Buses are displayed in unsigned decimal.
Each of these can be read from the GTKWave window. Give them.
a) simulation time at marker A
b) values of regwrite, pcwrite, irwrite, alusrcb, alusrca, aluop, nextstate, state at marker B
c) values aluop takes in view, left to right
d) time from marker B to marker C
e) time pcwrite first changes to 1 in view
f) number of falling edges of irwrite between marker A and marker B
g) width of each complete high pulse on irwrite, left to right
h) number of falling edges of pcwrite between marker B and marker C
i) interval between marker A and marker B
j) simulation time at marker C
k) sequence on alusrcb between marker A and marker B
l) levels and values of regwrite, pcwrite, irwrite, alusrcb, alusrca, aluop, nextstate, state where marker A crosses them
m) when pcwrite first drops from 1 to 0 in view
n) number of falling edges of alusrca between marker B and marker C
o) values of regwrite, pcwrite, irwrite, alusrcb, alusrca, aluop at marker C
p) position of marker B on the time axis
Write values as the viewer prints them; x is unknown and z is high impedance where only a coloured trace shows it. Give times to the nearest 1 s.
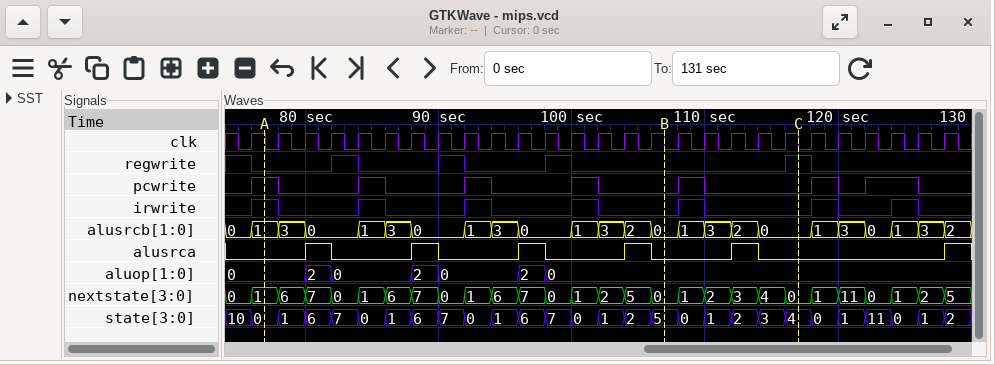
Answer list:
77 s
regwrite=0, pcwrite=0, irwrite=0, alusrcb=0, alusrca=0, aluop=0, nextstate=0, state=5
0, 2, 0, 2, 0, 2, 0
10 s
76 s
4
2 s, 2 s, 2 s, 2 s, 2 s, 2 s, 2 s
1
30 s
117 s
1, 3, 0, 1, 3, 0, 1, 3, 0, 1, 3, 2, 0
regwrite=0, pcwrite=1, irwrite=1, alusrcb=1, alusrca=0, aluop=0, nextstate=1, state=0
78 s
1
regwrite=1, pcwrite=0, irwrite=0, alusrcb=0, alusrca=0, aluop=0
107 s
